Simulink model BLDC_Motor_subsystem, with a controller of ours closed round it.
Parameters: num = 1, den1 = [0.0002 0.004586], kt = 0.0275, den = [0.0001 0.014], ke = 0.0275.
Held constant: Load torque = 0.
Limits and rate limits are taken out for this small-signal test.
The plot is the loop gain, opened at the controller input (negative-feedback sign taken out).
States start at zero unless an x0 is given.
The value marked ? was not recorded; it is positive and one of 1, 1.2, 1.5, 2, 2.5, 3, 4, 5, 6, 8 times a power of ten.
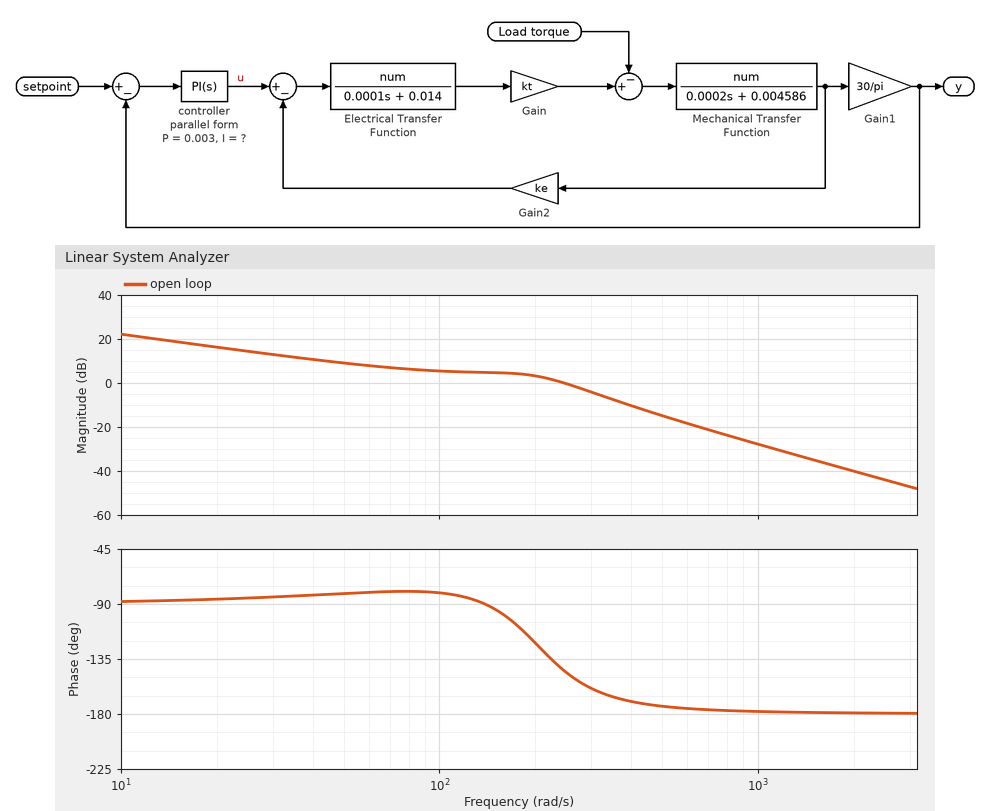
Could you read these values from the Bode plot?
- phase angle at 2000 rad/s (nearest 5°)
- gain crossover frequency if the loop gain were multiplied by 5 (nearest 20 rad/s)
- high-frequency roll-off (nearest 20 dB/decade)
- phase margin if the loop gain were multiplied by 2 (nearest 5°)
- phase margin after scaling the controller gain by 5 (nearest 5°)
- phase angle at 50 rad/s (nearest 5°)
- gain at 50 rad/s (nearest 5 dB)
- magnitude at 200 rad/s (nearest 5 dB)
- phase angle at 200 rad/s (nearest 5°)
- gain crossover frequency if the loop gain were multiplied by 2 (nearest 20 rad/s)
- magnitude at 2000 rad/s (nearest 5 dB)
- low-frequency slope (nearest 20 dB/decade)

-180°
480 rad/s
-40 dB/decade
15°
5°
-80°
10 dB
5 dB
-120°
320 rad/s
-40 dB
-20 dB/decade
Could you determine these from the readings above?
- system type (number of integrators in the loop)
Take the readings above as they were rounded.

1
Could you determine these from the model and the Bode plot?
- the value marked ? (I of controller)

0.4
